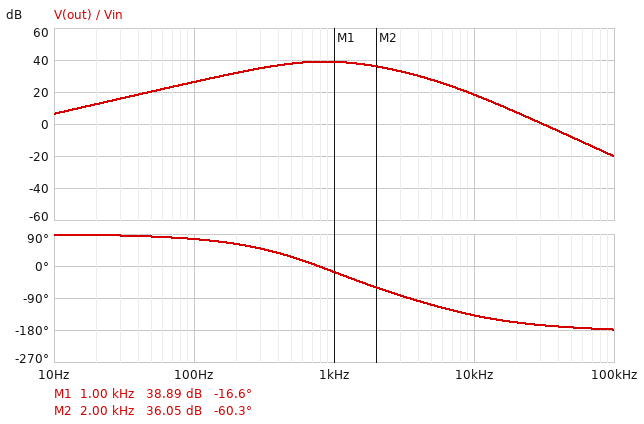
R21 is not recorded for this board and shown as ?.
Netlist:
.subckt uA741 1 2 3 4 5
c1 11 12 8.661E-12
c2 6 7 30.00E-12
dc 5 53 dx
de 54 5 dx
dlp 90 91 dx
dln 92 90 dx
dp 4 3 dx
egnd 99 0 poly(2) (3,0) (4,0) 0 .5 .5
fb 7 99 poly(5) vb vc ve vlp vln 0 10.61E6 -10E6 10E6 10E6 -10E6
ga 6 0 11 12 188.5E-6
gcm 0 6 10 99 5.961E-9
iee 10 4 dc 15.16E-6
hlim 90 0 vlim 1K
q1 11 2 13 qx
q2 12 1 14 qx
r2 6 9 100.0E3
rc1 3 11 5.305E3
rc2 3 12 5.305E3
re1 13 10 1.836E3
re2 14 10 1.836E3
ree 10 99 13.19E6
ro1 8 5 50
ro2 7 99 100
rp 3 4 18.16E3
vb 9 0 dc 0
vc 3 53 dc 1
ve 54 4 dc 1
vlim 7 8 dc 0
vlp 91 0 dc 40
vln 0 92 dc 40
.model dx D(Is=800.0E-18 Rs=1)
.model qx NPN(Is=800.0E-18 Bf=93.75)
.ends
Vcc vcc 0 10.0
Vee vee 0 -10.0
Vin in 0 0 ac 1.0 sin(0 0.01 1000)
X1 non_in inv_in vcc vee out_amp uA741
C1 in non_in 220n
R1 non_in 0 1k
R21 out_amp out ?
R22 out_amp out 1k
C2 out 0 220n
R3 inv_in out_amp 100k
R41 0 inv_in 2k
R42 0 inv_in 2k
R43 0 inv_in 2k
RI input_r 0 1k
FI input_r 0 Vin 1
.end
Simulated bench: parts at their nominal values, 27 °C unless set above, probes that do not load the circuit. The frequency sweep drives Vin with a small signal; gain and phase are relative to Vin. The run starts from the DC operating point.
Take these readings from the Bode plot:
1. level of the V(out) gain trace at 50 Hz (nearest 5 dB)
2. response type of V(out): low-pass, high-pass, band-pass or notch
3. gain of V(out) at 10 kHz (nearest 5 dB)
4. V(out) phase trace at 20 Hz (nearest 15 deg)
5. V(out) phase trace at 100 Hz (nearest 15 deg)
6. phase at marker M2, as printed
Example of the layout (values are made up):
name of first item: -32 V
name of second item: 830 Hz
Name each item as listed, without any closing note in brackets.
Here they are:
level of the V(out) gain trace at 50 Hz: 20 dB
response type of V(out): low-pass, high-pass, band-pass or notch: band-pass
gain of V(out) at 10 kHz: 20 dB
V(out) phase trace at 20 Hz: 90 deg
V(out) phase trace at 100 Hz: 75 deg
phase at marker M2, as printed: -60.3 deg
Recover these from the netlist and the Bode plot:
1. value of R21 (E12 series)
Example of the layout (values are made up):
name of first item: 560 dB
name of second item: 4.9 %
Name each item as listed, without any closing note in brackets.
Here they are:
value of R21: 2.2 kΩ
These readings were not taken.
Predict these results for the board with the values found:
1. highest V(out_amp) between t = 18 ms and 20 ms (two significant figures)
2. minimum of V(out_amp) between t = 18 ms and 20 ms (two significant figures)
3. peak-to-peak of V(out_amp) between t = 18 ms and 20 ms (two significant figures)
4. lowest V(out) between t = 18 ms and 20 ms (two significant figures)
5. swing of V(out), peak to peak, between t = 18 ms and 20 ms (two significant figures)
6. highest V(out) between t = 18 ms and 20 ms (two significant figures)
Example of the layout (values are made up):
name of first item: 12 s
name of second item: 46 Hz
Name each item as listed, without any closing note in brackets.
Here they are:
highest V(out_amp) between t = 18 ms and 20 ms: 1.2 V
minimum of V(out_amp) between t = 18 ms and 20 ms: -1.2 V
peak-to-peak of V(out_amp) between t = 18 ms and 20 ms: 2.4 V
lowest V(out) between t = 18 ms and 20 ms: -880 mV
swing of V(out), peak to peak, between t = 18 ms and 20 ms: 1.8 V
highest V(out) between t = 18 ms and 20 ms: 880 mV
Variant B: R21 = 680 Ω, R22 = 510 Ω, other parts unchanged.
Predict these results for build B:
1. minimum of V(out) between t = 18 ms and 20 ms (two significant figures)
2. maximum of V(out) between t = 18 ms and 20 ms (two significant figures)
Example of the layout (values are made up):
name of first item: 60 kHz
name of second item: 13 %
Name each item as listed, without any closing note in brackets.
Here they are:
minimum of V(out) between t = 18 ms and 20 ms: -1.1 V
maximum of V(out) between t = 18 ms and 20 ms: 1.1 V
